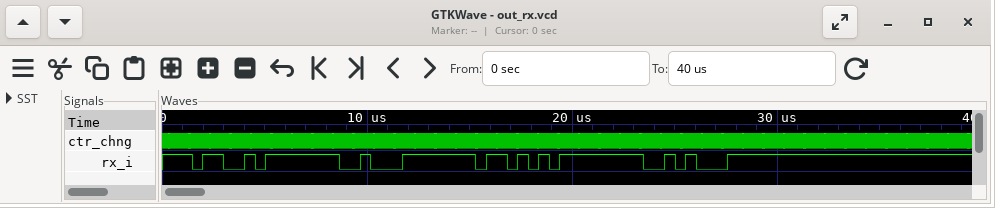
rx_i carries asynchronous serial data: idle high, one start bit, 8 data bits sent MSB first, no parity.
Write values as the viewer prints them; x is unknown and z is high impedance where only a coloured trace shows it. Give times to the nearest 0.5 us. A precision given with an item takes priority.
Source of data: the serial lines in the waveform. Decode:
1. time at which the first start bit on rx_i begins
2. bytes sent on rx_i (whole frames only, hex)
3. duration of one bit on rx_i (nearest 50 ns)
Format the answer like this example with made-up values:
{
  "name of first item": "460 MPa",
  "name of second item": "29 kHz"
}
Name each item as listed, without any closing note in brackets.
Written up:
{
  "time at which the first start bit on rx_i begins": "1.5 us",
  "bytes sent on rx_i": "CB, 47, D5, 51",
  "duration of one bit on rx_i": "500 ns"
}
